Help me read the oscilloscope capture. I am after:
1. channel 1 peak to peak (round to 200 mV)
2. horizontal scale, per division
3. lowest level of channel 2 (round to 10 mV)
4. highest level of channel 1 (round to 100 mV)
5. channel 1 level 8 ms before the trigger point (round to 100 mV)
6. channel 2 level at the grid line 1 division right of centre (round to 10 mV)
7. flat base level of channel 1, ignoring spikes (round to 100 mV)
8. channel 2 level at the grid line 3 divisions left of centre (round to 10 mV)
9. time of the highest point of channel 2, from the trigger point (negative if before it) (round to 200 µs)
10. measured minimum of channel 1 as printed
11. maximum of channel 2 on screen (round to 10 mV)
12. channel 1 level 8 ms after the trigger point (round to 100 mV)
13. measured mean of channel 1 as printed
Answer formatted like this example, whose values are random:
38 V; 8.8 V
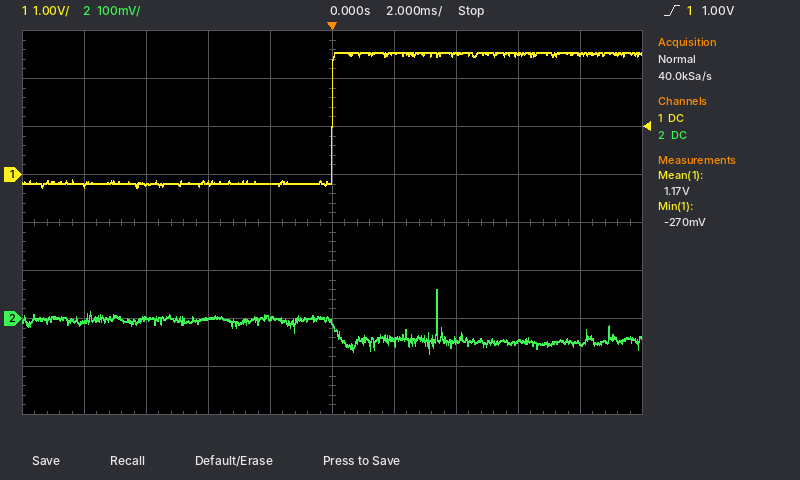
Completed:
2.8 V; 2 ms; -70 mV; 2.5 V; -200 mV; -50 mV; -200 mV; 0 mV; +3.4 ms; -270 mV; 60 mV; 2.5 V; 1.17 V
